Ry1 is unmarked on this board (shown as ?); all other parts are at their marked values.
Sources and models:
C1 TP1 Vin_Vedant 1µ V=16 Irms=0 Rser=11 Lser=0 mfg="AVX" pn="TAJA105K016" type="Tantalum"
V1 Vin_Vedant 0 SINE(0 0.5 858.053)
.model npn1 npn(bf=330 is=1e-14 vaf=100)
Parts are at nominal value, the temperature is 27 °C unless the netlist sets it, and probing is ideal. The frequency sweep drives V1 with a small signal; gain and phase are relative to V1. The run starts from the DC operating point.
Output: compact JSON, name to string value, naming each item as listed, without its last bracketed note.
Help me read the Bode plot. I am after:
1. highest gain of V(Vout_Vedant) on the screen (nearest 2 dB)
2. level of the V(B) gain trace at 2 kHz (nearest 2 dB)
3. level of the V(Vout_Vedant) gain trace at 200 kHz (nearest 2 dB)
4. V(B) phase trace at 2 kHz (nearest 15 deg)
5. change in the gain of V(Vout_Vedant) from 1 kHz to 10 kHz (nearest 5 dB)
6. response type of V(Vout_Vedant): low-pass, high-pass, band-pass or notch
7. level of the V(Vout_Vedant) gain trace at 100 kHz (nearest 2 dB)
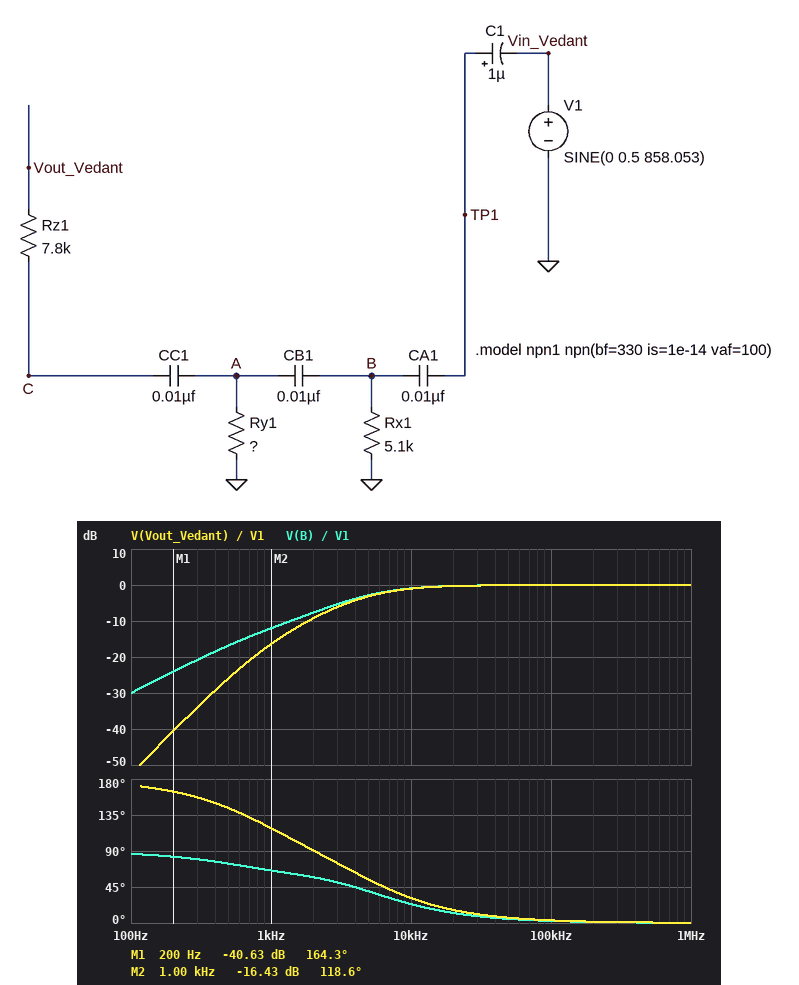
{"highest gain of V(Vout_Vedant) on the screen": "0 dB", "level of the V(B) gain trace at 2 kHz": "-8 dB", "level of the V(Vout_Vedant) gain trace at 200 kHz": "0 dB", "V(B) phase trace at 2 kHz": "60 deg", "change in the gain of V(Vout_Vedant) from 1 kHz to 10 kHz": "15 dB", "response type of V(Vout_Vedant): low-pass, high-pass, band-pass or notch": "high-pass", "level of the V(Vout_Vedant) gain trace at 100 kHz": "0 dB"}
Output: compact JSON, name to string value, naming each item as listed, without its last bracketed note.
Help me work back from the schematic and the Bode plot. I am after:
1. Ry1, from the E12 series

{"Ry1, from the E12 series": "12 kΩ"}
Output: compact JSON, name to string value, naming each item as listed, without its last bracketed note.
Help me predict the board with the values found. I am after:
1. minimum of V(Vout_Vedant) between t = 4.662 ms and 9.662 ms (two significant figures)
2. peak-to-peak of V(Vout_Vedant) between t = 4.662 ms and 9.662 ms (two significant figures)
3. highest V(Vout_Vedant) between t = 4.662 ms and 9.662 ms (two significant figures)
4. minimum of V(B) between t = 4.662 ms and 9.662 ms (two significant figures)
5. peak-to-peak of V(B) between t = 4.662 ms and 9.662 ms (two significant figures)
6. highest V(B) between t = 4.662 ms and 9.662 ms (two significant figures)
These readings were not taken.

{"minimum of V(Vout_Vedant) between t = 4.662 ms and 9.662 ms": "-61 mV", "peak-to-peak of V(Vout_Vedant) between t = 4.662 ms and 9.662 ms": "120 mV", "highest V(Vout_Vedant) between t = 4.662 ms and 9.662 ms": "61 mV", "minimum of V(B) between t = 4.662 ms and 9.662 ms": "-110 mV", "peak-to-peak of V(B) between t = 4.662 ms and 9.662 ms": "220 mV", "highest V(B) between t = 4.662 ms and 9.662 ms": "110 mV"}
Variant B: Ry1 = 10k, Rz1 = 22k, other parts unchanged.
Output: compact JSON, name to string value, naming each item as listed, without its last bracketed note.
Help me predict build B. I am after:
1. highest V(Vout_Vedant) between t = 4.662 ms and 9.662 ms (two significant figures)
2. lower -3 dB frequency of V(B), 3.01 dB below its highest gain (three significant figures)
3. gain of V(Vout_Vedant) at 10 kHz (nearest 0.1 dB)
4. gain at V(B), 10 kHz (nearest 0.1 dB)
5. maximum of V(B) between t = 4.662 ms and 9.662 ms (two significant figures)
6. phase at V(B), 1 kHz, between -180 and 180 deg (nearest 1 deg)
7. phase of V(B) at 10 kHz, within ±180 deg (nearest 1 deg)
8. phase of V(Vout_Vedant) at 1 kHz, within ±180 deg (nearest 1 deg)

{"highest V(Vout_Vedant) between t = 4.662 ms and 9.662 ms": "53 mV", "lower -3 dB frequency of V(B), 3.01 dB below its highest gain": "5.10 kHz", "gain of V(Vout_Vedant) at 10 kHz": "-1.2 dB", "gain at V(B), 10 kHz": "-1.1 dB", "maximum of V(B) between t = 4.662 ms and 9.662 ms": "110 mV", "phase at V(B), 1 kHz, between -180 and 180 deg": "64 deg", "phase of V(B) at 10 kHz, within ±180 deg": "25 deg", "phase of V(Vout_Vedant) at 1 kHz, within ±180 deg": "122 deg"}
